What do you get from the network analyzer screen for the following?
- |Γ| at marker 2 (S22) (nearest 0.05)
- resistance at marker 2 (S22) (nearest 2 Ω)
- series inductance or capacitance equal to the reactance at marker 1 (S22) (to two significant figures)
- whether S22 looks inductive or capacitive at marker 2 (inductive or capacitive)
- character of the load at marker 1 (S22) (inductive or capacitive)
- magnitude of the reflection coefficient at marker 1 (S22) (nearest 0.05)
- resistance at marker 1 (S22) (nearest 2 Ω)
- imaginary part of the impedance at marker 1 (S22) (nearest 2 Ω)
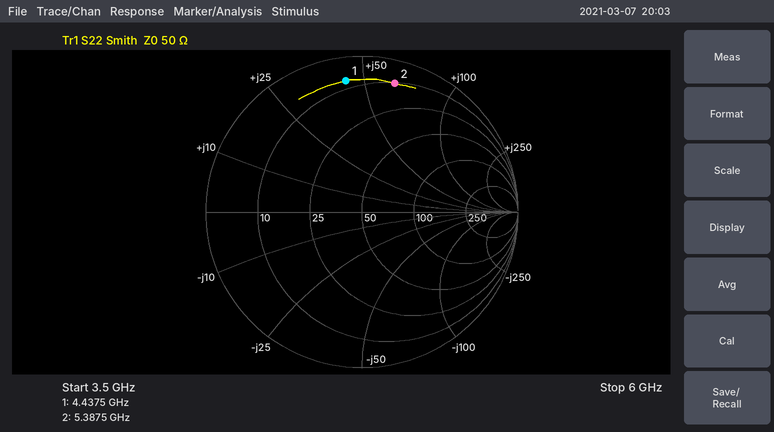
0.85
10 Ω
1.6 nH
inductive
inductive
0.85
8 Ω
+44 Ω
